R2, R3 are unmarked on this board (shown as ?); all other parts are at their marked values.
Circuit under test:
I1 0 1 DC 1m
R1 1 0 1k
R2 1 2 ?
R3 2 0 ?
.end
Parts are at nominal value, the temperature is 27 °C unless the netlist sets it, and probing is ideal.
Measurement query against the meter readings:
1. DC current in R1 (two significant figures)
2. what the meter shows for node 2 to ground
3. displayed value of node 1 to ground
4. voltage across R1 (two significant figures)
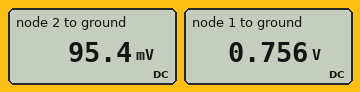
760 µA
95.4 mV
0.756 V
760 mV
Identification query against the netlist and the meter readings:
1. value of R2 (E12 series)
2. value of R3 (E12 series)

2.7 kΩ
390 Ω
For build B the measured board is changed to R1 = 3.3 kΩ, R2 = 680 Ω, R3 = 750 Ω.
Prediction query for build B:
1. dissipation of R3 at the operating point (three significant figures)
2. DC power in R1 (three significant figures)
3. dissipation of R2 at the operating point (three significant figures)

365 µW
302 µW
331 µW
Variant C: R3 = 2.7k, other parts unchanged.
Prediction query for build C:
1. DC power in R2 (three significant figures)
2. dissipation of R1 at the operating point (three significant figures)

65.9 µW
712 µW
